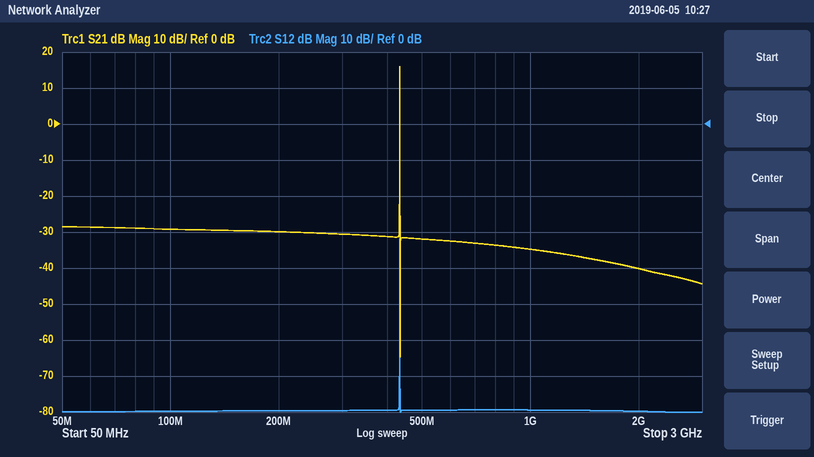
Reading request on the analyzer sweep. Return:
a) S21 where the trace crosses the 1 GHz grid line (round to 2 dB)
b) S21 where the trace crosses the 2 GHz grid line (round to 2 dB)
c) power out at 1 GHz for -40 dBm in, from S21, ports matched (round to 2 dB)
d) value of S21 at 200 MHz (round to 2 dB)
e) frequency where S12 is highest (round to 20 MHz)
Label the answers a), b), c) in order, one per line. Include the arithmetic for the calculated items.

a) -34 dB
b) -40 dB
c) -40 dBm + (-34 dB) = -74 dBm
d) -30 dB
e) 440 MHz
